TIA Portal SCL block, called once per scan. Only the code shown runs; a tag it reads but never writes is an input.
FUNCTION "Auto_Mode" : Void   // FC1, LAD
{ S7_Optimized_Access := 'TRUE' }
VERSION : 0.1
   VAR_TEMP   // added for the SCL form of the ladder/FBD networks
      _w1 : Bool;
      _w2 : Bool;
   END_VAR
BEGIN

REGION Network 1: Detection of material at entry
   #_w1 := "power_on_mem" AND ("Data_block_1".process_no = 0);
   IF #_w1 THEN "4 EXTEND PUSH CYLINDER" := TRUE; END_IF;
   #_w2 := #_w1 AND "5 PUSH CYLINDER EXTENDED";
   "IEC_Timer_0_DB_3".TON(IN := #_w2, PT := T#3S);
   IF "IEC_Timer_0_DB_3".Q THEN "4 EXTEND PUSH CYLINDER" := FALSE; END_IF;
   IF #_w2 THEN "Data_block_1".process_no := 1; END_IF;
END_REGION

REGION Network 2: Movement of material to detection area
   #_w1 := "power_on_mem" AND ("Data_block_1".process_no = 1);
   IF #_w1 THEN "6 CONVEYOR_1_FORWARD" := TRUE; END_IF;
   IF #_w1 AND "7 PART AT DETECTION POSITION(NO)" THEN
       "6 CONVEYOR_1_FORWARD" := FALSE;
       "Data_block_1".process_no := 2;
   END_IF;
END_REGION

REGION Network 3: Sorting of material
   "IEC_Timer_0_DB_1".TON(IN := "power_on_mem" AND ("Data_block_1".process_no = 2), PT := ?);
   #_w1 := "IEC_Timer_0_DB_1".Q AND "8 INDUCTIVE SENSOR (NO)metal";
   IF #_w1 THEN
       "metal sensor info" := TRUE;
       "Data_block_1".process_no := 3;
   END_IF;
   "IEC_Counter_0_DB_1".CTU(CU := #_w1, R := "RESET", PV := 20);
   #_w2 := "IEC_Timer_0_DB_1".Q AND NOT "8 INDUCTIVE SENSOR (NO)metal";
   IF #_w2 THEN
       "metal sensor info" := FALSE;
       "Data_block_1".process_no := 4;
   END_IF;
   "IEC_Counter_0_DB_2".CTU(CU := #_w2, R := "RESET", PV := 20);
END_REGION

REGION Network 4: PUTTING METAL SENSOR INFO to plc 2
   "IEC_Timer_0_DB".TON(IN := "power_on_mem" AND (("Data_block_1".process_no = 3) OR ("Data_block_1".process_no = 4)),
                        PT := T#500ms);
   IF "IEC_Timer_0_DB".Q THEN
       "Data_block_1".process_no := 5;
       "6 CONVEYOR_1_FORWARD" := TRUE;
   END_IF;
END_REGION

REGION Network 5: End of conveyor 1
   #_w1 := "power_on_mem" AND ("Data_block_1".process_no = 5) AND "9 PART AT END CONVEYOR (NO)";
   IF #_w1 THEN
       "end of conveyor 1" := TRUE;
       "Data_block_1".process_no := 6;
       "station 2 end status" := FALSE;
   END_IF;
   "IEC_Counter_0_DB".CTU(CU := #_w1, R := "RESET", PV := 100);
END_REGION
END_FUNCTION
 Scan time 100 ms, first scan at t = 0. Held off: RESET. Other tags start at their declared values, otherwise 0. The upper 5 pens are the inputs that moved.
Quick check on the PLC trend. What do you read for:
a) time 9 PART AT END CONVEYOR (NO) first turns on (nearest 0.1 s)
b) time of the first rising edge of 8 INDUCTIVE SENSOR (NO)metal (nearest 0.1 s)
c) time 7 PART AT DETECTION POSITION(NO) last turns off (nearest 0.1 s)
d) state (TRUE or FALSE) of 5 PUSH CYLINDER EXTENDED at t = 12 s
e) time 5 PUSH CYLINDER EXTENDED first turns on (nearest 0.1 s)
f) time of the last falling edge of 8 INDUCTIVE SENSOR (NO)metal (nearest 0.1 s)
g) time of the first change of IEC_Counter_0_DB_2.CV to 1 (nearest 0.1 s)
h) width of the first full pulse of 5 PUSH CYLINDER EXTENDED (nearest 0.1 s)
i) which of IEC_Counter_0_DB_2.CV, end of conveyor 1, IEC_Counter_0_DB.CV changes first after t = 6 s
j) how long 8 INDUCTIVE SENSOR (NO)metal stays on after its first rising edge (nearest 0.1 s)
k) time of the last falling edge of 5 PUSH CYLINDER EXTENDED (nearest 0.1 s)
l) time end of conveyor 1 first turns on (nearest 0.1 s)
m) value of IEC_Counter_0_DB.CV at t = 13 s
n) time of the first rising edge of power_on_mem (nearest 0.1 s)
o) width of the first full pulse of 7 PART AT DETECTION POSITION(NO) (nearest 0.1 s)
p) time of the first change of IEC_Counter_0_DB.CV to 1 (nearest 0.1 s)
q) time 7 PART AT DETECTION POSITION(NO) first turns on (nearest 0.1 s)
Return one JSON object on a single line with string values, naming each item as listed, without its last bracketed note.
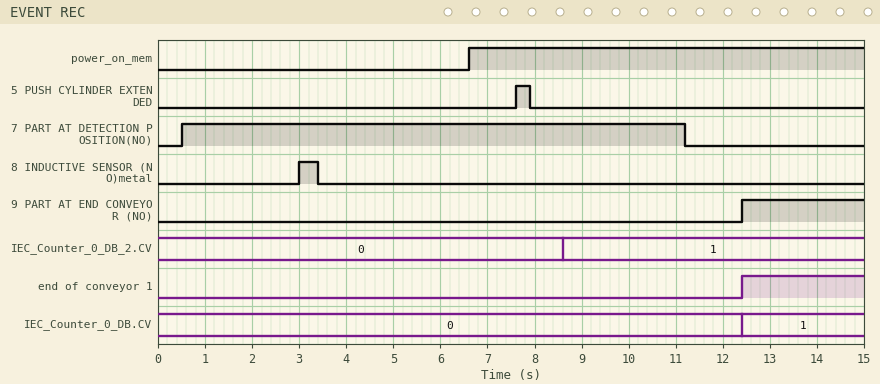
{"time 9 PART AT END CONVEYOR (NO) first turns on": "12.4 s", "time of the first rising edge of 8 INDUCTIVE SENSOR (NO)metal": "3.0 s", "time 7 PART AT DETECTION POSITION(NO) last turns off": "11.2 s", "state (TRUE or FALSE) of 5 PUSH CYLINDER EXTENDED at t = 12 s": "FALSE", "time 5 PUSH CYLINDER EXTENDED first turns on": "7.6 s", "time of the last falling edge of 8 INDUCTIVE SENSOR (NO)metal": "3.4 s", "time of the first change of IEC_Counter_0_DB_2.CV to 1": "8.6 s", "width of the first full pulse of 5 PUSH CYLINDER EXTENDED": "0.3 s", "which of IEC_Counter_0_DB_2.CV, end of conveyor 1, IEC_Counter_0_DB.CV changes first after t = 6 s": "IEC_Counter_0_DB_2.CV", "how long 8 INDUCTIVE SENSOR (NO)metal stays on after its first rising edge": "0.4 s", "time of the last falling edge of 5 PUSH CYLINDER EXTENDED": "7.9 s", "time end of conveyor 1 first turns on": "12.4 s", "value of IEC_Counter_0_DB.CV at t = 13 s": "1", "time of the first rising edge of power_on_mem": "6.6 s", "width of the first full pulse of 7 PART AT DETECTION POSITION(NO)": "10.7 s", "time of the first change of IEC_Counter_0_DB.CV to 1": "12.4 s", "time 7 PART AT DETECTION POSITION(NO) first turns on": "0.5 s"}
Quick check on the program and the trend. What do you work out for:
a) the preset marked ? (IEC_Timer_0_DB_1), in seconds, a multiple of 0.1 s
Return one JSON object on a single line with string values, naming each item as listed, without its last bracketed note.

{"the preset marked ? (IEC_Timer_0_DB_1), in seconds, a multiple of 0.1 s": "1.0 s"}
